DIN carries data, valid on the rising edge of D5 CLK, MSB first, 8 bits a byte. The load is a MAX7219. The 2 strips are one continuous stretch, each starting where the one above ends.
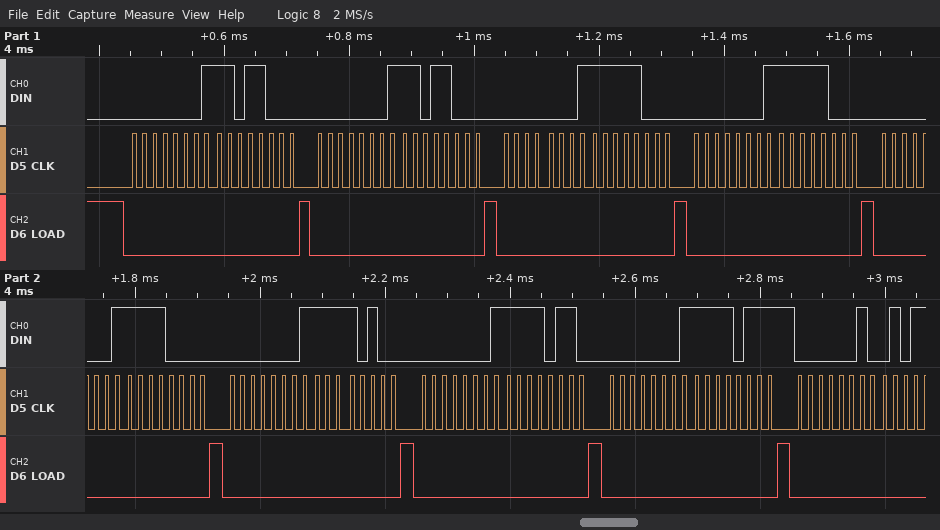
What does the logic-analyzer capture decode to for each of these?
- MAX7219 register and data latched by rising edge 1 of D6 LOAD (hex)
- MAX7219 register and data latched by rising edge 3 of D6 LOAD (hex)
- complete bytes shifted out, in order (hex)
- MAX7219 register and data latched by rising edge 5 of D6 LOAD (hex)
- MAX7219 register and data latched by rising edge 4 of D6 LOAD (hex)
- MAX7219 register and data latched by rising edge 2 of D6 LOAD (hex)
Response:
register 0x1, data 0xD8
register 0x1, data 0xF8
01 D8 01 D8 01 F8 01 F8 01 F0 01 F4 01 F6 01 F7 02
register 0x1, data 0xF0
register 0x1, data 0xF8
register 0x1, data 0xD8
